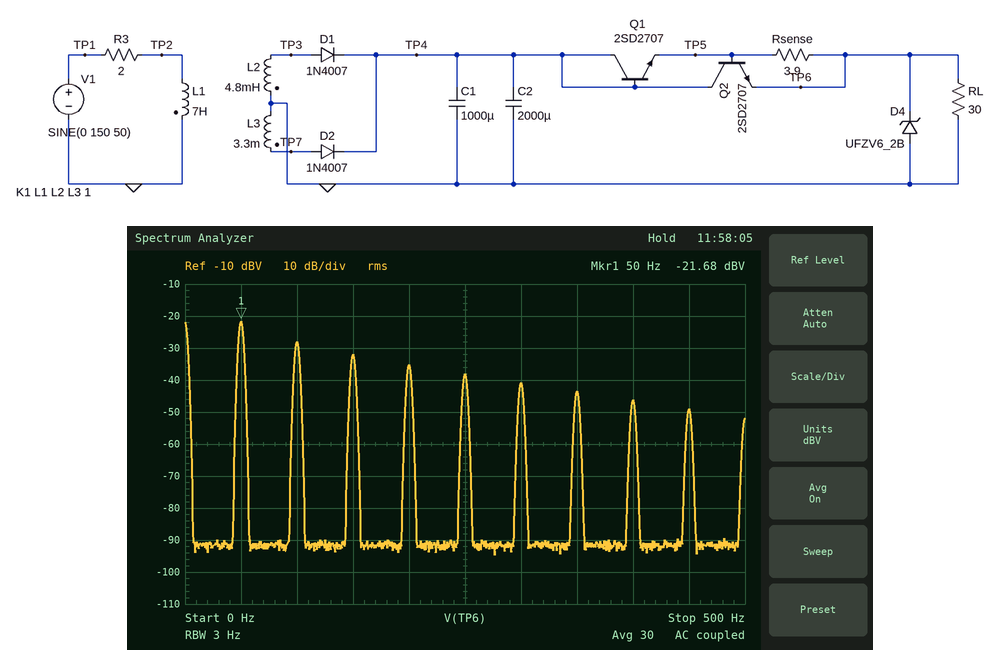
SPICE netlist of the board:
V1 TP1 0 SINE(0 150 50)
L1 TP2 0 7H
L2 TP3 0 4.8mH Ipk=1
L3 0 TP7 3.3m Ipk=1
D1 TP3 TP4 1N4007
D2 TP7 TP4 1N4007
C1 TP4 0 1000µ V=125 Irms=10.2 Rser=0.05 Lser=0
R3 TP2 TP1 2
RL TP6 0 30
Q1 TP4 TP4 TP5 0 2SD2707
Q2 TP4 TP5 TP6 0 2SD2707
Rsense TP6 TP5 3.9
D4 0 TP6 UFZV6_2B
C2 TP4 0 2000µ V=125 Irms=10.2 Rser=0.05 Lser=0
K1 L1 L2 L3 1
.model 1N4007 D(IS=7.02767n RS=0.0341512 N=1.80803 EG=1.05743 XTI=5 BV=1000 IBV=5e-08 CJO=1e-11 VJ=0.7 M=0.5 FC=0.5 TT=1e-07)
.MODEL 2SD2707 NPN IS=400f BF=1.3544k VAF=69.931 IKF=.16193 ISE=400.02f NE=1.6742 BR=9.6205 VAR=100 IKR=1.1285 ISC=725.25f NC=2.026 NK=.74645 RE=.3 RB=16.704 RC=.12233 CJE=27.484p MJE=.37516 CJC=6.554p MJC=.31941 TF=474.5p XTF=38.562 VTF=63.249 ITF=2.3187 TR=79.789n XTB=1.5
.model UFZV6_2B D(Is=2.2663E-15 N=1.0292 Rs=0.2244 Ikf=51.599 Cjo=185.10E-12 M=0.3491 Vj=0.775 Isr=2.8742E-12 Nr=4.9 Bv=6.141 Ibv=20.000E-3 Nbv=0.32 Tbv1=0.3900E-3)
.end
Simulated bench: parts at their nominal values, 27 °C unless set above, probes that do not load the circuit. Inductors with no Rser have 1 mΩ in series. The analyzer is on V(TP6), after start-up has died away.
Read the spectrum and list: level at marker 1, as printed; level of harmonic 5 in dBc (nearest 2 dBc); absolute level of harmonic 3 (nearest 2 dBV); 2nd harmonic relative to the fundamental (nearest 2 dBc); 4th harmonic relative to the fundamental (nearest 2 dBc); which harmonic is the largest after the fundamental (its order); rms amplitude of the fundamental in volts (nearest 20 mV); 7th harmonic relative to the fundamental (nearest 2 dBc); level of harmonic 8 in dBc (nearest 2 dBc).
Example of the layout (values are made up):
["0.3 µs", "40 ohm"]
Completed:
["-21.68 dBV", "-16 dBc", "-32 dBV", "-6 dBc", "-14 dBc", "2", "80 mV", "-22 dBc", "-24 dBc"]
